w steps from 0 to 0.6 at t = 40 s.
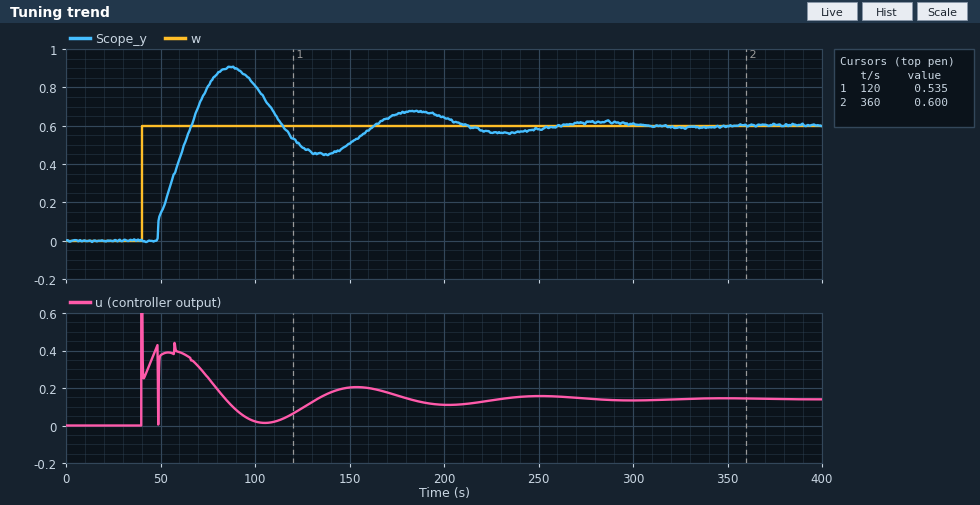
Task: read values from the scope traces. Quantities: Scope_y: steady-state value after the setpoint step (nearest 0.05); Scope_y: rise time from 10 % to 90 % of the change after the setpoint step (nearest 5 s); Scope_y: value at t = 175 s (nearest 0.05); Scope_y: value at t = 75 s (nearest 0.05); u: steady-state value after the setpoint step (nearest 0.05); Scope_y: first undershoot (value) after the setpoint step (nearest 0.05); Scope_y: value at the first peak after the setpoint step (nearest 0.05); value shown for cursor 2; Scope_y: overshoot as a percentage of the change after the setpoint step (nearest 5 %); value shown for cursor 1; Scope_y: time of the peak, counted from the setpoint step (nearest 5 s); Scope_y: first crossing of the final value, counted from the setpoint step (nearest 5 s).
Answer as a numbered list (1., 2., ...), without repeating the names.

1. 0.60
2. 15 s
3. 0.65
4. 0.80
5. 0.15
6. 0.45
7. 0.90
8. 0.600
9. 50 %
10. 0.535
11. 45 s
12. 25 s
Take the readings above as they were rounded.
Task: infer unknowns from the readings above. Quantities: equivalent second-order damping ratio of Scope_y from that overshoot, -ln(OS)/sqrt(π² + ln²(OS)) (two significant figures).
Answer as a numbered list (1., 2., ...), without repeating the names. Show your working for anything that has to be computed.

1. ln(0.5) = -0.693; 0.693 / sqrt(9.870 + 0.480) = 0.22
